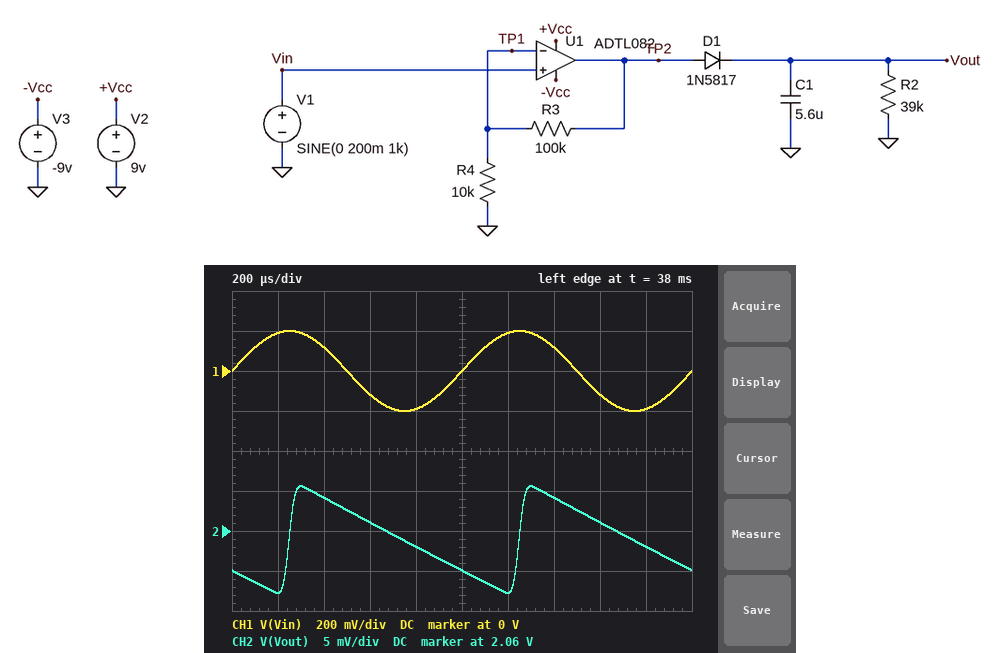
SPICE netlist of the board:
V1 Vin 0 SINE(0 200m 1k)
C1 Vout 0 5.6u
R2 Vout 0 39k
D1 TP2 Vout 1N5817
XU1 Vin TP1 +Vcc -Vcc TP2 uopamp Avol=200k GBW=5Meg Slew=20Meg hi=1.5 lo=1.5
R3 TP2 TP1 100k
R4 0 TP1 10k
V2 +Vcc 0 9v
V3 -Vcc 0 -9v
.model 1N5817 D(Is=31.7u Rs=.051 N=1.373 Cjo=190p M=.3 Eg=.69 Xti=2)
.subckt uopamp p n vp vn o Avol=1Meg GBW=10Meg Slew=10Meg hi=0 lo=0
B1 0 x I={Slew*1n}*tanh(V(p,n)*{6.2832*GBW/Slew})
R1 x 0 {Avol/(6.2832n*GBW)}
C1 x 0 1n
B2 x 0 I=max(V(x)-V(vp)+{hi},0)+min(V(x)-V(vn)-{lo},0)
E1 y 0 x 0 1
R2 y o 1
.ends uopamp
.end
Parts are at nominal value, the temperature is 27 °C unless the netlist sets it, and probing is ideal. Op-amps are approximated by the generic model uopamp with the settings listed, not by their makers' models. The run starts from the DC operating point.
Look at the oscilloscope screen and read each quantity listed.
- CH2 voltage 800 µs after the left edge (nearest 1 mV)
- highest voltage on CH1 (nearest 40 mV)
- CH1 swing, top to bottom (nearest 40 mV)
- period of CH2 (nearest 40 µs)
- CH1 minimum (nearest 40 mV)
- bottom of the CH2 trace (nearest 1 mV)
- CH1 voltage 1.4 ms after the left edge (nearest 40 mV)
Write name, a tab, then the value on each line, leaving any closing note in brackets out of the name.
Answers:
CH2 voltage 800 µs after the left edge	2.058 V
highest voltage on CH1	200 mV
CH1 swing, top to bottom	400 mV
period of CH2	1.00 ms
CH1 minimum	-200 mV
bottom of the CH2 trace	2.052 V
CH1 voltage 1.4 ms after the left edge	120 mV
